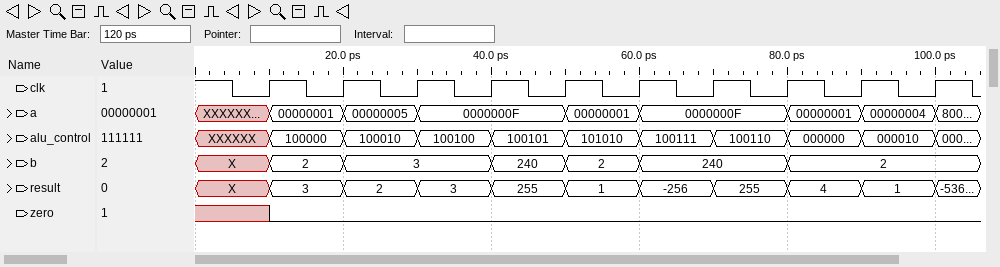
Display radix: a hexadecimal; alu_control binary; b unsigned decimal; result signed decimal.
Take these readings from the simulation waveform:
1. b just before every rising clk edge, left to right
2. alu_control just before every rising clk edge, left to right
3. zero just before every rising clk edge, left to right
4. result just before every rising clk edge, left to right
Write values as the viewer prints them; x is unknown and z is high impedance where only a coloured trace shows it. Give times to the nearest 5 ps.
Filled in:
X, 2, 3, 3, 240, 2, 240, 240, 2, 2
XXXXXX, 100000, 100010, 100100, 100101, 101010, 100111, 100110, 000000, 000010
x 0 0 0 0 0 0 0 0 0
X, 3, 2, 3, 255, 1, -256, 255, 4, 1
